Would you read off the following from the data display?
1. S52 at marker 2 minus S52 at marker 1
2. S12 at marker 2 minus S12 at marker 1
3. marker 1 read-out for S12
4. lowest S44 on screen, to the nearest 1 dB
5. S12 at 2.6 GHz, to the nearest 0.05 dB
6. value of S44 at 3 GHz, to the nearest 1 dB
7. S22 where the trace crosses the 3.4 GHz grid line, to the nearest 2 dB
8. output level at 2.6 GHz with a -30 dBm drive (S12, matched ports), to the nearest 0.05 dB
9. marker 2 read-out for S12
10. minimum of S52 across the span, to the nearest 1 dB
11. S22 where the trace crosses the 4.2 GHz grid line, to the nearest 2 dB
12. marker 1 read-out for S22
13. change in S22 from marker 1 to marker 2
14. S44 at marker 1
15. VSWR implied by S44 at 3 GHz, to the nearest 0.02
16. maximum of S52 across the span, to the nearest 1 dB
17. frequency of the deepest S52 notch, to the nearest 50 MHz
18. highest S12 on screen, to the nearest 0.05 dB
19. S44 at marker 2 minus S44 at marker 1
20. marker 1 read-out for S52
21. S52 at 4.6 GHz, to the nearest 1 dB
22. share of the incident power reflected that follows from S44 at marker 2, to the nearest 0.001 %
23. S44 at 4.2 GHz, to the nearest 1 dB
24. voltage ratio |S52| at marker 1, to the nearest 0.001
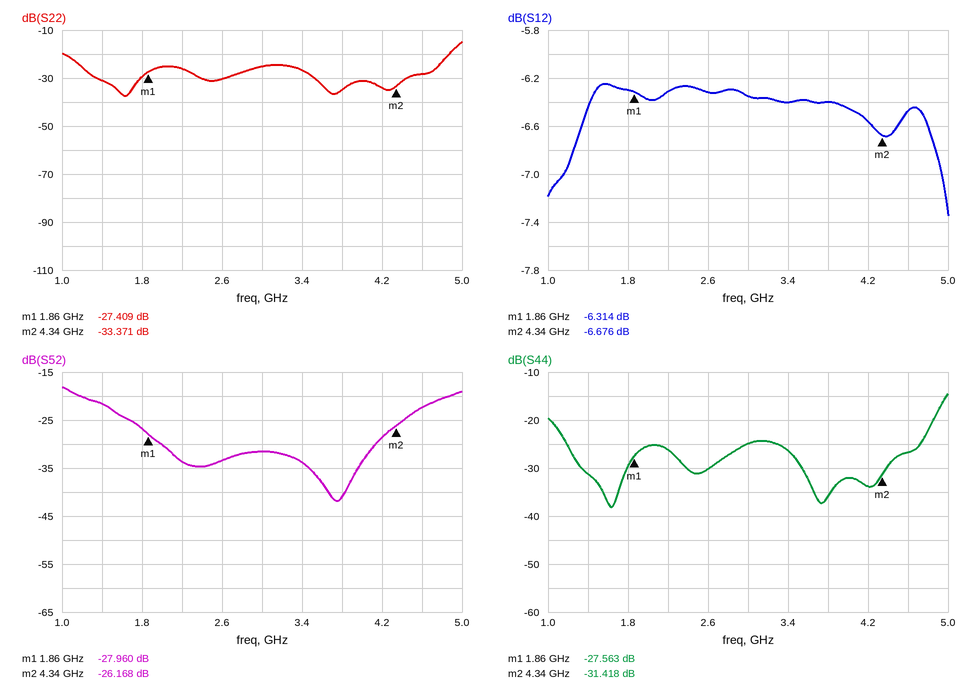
1.792 dB
-0.362 dB
-6.314 dB
-38 dB
-6.30 dB
-25 dB
-26 dB
-36.30 dBm
-6.676 dB
-42 dB
-34 dB
-27.409 dB
-5.962 dB
-27.563 dB
1.12
-18 dB
3.75 GHz
-6.25 dB
-3.855 dB
-27.960 dB
-22 dB
0.072 %
-34 dB
0.040
